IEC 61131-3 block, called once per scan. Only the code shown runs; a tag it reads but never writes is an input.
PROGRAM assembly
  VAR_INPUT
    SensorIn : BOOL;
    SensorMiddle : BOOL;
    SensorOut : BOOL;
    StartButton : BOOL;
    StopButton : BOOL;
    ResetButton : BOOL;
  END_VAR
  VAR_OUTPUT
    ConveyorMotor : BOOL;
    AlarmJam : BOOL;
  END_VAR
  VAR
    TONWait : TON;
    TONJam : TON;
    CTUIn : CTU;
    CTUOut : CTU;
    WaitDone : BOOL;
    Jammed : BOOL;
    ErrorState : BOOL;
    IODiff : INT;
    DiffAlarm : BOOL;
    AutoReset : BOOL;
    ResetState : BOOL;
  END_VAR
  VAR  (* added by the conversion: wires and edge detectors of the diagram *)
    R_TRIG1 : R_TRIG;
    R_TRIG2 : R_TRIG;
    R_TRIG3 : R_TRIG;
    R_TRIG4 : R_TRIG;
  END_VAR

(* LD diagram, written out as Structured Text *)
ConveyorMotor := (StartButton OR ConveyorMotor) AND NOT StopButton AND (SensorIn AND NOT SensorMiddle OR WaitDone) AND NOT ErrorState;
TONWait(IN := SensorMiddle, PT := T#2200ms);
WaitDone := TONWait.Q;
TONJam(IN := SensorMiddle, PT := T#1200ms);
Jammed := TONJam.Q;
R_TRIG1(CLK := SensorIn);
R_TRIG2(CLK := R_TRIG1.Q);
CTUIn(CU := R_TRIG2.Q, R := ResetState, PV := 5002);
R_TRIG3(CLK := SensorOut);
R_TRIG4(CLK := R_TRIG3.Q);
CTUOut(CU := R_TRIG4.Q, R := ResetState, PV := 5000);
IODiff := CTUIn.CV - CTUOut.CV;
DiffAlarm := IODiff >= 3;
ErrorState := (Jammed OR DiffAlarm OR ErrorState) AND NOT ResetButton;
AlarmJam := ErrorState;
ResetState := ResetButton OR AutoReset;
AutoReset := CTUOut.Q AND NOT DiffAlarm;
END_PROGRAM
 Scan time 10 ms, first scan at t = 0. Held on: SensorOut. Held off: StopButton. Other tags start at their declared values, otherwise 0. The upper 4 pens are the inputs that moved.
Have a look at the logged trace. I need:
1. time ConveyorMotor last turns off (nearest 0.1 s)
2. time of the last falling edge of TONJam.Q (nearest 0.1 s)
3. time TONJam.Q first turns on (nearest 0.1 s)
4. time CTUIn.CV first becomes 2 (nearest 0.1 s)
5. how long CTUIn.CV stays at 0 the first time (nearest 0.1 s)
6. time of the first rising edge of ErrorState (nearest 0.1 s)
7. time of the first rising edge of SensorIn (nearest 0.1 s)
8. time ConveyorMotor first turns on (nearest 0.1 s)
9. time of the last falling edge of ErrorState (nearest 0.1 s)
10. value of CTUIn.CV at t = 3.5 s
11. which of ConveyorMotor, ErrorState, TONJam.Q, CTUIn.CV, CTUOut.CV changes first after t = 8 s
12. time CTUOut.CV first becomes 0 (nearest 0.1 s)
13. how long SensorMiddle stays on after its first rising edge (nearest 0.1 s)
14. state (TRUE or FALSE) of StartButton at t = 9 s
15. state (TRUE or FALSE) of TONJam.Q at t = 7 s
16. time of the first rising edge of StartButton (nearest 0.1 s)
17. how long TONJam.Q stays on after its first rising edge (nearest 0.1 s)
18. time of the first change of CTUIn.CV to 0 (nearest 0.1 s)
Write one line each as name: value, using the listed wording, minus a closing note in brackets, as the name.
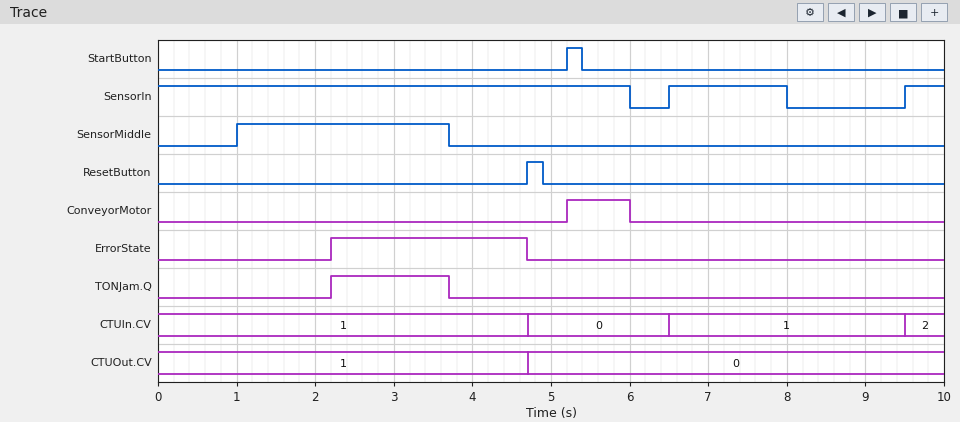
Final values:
time ConveyorMotor last turns off: 6.0 s
time of the last falling edge of TONJam.Q: 3.7 s
time TONJam.Q first turns on: 2.2 s
time CTUIn.CV first becomes 2: 9.5 s
how long CTUIn.CV stays at 0 the first time: 1.8 s
time of the first rising edge of ErrorState: 2.2 s
time of the first rising edge of SensorIn: 6.5 s
time ConveyorMotor first turns on: 5.2 s
time of the last falling edge of ErrorState: 4.7 s
value of CTUIn.CV at t = 3.5 s: 1
which of ConveyorMotor, ErrorState, TONJam.Q, CTUIn.CV, CTUOut.CV changes first after t = 8 s: CTUIn.CV
time CTUOut.CV first becomes 0: 4.7 s
how long SensorMiddle stays on after its first rising edge: 2.7 s
state (TRUE or FALSE) of StartButton at t = 9 s: FALSE
state (TRUE or FALSE) of TONJam.Q at t = 7 s: FALSE
time of the first rising edge of StartButton: 5.2 s
how long TONJam.Q stays on after its first rising edge: 1.5 s
time of the first change of CTUIn.CV to 0: 4.7 s
